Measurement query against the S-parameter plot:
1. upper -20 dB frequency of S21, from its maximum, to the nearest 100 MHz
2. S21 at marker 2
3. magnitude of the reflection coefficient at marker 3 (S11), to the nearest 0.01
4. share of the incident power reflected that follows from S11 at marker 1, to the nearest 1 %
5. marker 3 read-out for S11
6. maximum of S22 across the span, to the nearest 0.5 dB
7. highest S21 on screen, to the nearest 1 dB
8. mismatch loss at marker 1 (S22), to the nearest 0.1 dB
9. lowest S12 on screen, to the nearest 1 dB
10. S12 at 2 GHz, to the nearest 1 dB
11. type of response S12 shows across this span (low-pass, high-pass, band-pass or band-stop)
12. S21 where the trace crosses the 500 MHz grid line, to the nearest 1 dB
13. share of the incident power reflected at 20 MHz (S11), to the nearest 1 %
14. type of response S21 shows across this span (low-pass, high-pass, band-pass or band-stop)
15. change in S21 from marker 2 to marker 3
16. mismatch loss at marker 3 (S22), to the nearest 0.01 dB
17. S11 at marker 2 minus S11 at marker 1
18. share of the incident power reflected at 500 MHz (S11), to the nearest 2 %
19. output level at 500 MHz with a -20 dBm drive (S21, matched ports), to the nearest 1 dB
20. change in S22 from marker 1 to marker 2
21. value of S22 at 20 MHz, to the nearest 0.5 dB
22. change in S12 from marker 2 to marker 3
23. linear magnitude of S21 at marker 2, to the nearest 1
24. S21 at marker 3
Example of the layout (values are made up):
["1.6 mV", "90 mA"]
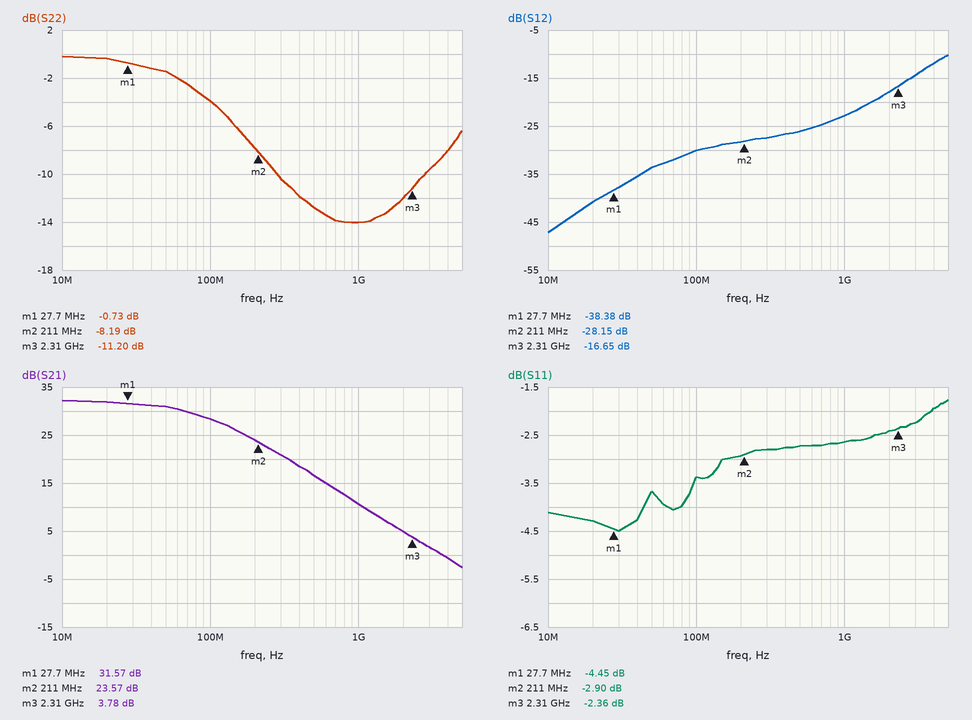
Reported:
["800 MHz", "23.57 dB", "0.76", "36 %", "-2.36 dB", "0.0 dB", "32 dB", "8.1 dB", "-47 dB", "-18 dB", "high-pass", "17 dB", "37 %", "low-pass", "-19.79 dB", "0.34 dB", "1.55 dB", "54 %", "-3 dBm", "-7.46 dB", "-0.5 dB", "11.50 dB", "15", "3.78 dB"]
